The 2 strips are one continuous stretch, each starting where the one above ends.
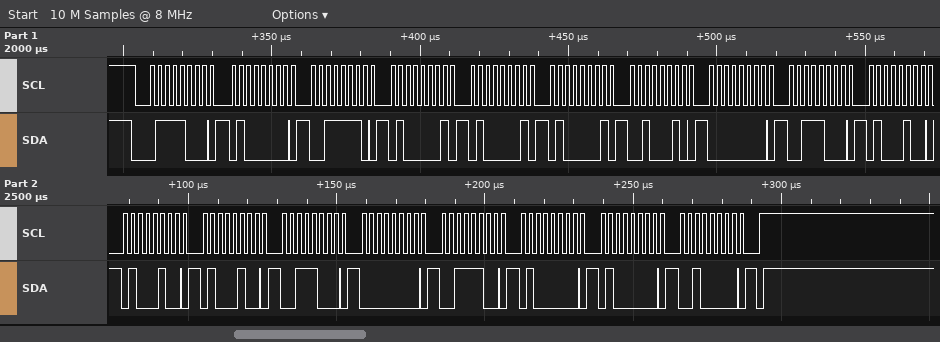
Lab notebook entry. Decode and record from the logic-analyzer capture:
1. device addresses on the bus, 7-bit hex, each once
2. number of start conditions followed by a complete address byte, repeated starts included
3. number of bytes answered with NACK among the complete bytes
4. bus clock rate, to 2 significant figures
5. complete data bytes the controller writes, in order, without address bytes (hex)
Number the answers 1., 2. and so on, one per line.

1. 0x3C
2. 1
3. 0
4. 400 kHz
5. 40 3E 41 41 41 22 00 38 44 44 44 38 00 3C 40 40 20
